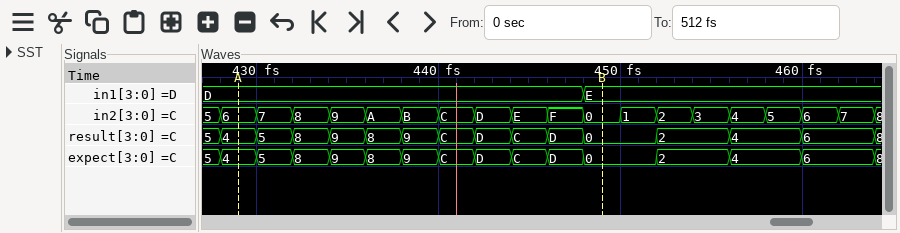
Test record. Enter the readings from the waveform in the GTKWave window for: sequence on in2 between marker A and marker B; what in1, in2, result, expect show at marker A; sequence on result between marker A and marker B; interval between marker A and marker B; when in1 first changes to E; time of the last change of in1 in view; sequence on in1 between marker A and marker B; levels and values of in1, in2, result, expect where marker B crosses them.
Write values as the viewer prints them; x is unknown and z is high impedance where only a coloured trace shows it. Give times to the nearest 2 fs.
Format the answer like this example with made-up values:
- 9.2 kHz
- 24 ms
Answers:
- 6, 7, 8, 9, A, B, C, D, E, F, 0
- in1=D, in2=6, result=4, expect=4
- 4, 5, 8, 9, 8, 9, C, D, C, D, 0
- 20 fs
- 448 fs
- 448 fs
- D, E
- in1=E, in2=0, result=0, expect=0
